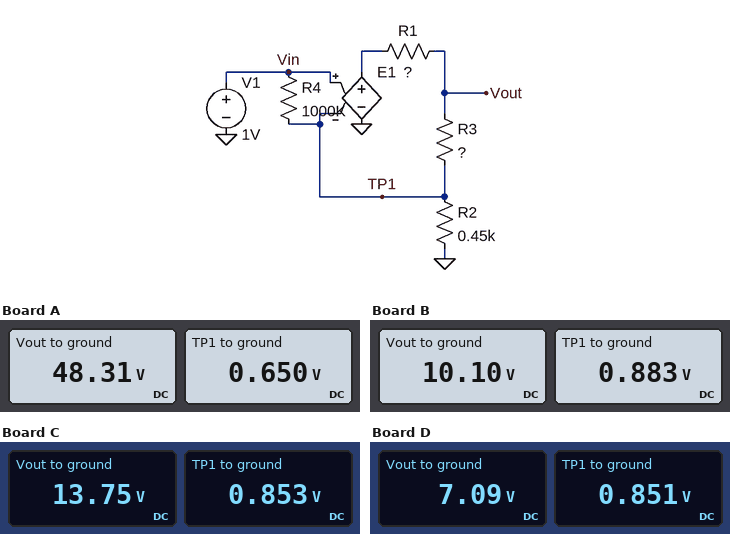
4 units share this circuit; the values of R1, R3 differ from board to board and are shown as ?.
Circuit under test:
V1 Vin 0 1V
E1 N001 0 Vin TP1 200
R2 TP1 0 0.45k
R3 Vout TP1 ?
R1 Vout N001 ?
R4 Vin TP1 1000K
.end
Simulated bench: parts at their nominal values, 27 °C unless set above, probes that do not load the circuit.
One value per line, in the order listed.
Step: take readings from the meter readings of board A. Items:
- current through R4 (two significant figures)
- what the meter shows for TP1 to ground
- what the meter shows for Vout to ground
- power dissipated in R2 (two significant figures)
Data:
350 nA
0.650 V
48.31 V
940 µW
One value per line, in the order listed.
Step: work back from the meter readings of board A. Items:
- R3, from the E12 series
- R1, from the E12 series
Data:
33 kΩ
15 kΩ
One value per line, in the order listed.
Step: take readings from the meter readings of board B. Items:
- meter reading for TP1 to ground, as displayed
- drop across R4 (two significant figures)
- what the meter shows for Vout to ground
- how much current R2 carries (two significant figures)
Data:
0.883 V
120 mV
10.10 V
2.0 mA
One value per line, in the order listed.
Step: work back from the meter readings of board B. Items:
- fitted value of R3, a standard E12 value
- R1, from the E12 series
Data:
4.7 kΩ
6.8 kΩ
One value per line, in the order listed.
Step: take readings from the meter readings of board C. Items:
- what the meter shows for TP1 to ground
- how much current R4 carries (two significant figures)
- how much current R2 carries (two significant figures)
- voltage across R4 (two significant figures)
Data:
0.853 V
150 nA
1.9 mA
150 mV
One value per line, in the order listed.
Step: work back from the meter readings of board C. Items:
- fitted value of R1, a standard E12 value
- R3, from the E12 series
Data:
8.2 kΩ
6.8 kΩ
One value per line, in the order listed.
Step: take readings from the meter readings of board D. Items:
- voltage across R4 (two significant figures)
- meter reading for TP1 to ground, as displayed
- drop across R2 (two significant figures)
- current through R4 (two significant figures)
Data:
150 mV
0.851 V
850 mV
150 nA
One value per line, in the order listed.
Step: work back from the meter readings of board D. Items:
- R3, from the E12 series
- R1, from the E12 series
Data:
3.3 kΩ
12 kΩ
